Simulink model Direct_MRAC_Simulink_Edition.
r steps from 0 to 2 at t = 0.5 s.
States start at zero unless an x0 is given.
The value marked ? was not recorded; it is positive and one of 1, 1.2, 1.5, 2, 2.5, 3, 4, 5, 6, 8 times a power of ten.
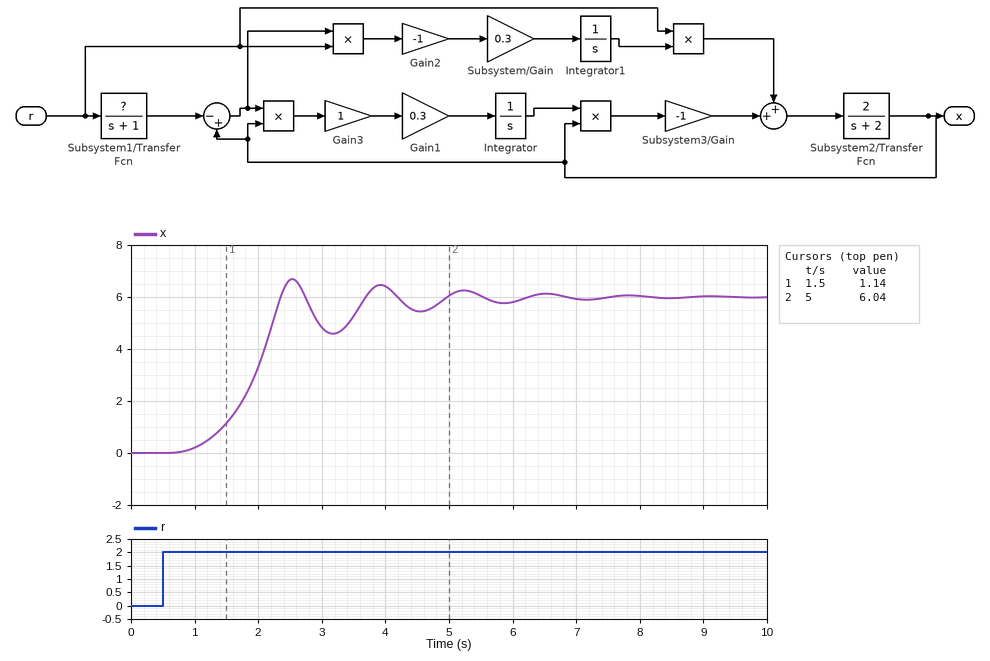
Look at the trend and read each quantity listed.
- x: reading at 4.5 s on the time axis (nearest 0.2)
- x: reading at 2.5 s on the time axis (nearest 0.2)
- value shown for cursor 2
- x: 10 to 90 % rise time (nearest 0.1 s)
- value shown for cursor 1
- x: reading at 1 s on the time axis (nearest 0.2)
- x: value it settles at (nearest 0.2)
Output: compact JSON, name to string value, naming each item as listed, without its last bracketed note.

{"x: reading at 4.5 s on the time axis": "5.4", "x: reading at 2.5 s on the time axis": "6.6", "value shown for cursor 2": "6.04", "x: 10 to 90 % rise time": "1.0 s", "value shown for cursor 1": "1.14", "x: reading at 1 s on the time axis": "0.2", "x: value it settles at": "6.0"}
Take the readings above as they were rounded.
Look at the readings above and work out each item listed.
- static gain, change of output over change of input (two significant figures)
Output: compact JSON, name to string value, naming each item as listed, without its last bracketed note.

{"static gain, change of output over change of input": "3.0"}
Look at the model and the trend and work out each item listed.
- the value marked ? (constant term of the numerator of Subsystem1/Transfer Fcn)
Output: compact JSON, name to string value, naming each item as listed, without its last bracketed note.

{"the value marked ?": "3"}
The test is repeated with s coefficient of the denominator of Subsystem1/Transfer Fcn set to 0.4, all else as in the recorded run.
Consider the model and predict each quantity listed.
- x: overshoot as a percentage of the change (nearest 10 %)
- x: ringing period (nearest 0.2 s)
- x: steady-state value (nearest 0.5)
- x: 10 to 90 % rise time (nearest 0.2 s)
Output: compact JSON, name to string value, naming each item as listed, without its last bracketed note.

{"x: overshoot as a percentage of the change": "40 %", "x: ringing period": "1.4 s", "x: steady-state value": "6.0", "x: 10 to 90 % rise time": "0.8 s"}
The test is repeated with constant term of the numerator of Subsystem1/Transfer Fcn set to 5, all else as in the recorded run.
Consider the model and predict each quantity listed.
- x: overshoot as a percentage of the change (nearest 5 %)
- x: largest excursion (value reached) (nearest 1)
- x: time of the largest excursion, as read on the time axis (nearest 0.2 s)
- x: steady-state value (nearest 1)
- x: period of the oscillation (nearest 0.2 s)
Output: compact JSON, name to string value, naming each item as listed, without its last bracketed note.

{"x: overshoot as a percentage of the change": "15 %", "x: largest excursion (value reached)": "11", "x: time of the largest excursion, as read on the time axis": "3.0 s", "x: steady-state value": "10", "x: period of the oscillation": "1.0 s"}
